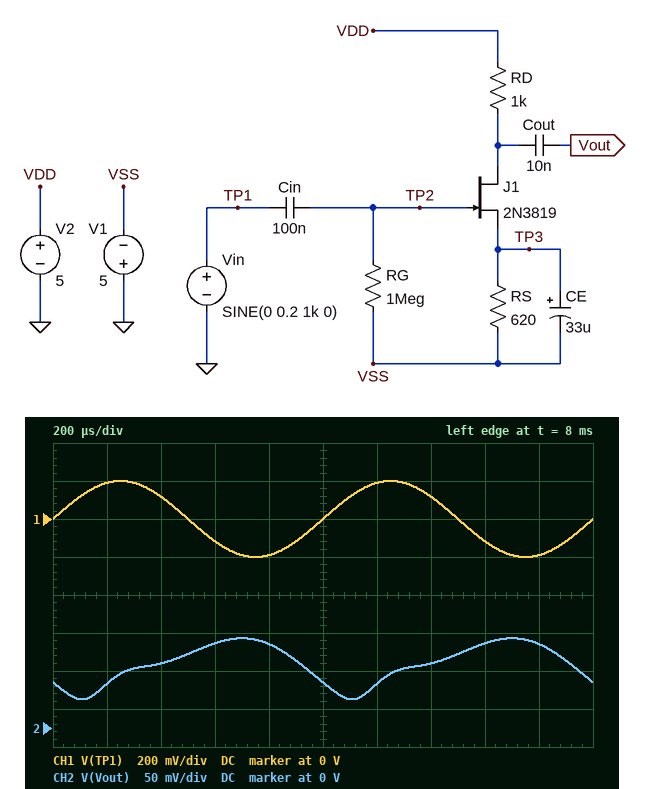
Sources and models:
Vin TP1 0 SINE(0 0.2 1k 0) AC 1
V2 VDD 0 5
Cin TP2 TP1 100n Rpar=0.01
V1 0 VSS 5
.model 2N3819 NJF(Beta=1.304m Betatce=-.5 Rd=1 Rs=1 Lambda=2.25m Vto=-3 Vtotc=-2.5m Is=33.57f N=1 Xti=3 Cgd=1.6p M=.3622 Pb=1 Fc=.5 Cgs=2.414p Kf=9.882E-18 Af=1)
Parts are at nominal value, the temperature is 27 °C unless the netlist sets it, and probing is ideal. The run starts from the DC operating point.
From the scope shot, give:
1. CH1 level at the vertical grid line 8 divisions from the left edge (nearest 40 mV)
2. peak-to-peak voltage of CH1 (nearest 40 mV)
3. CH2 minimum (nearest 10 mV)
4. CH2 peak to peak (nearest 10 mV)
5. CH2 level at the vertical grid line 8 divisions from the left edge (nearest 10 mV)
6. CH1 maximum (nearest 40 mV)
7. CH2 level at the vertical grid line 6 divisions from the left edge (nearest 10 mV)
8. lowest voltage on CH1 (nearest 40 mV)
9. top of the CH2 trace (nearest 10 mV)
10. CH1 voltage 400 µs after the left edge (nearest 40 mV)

-120 mV
400 mV
40 mV
80 mV
110 mV
200 mV
60 mV
-200 mV
120 mV
120 mV
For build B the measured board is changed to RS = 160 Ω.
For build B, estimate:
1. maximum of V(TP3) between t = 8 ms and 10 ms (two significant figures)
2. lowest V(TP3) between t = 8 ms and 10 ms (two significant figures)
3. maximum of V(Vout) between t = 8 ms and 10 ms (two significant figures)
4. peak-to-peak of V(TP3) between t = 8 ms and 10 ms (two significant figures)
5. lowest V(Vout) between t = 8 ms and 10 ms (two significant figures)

-550 mV
-860 mV
43 mV
310 mV
-240 mV
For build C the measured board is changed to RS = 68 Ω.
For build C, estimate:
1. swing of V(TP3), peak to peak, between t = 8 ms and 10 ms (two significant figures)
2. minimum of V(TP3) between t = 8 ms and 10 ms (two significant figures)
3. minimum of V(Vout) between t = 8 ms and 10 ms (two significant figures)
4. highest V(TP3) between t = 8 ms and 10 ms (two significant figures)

370 mV
-980 mV
-320 mV
-600 mV
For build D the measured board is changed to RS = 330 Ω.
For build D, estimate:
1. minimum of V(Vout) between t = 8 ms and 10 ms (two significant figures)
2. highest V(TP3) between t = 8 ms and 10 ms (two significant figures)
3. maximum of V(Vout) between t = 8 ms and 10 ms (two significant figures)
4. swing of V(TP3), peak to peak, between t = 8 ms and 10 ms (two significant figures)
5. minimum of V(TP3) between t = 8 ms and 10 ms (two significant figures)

-82 mV
-520 mV
60 mV
160 mV
-670 mV
